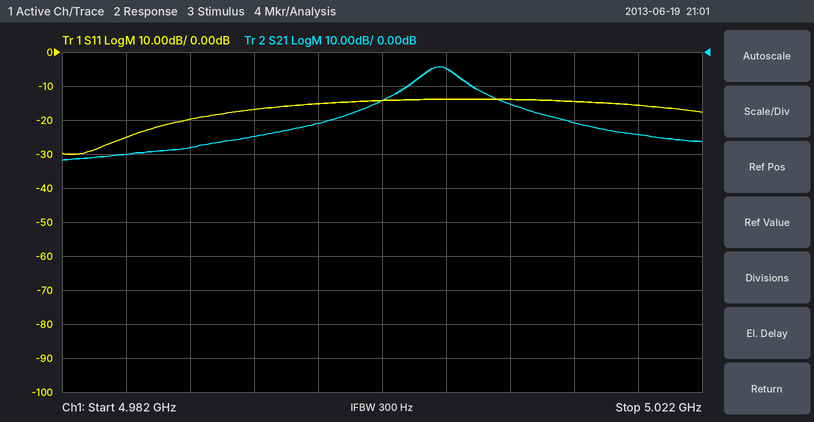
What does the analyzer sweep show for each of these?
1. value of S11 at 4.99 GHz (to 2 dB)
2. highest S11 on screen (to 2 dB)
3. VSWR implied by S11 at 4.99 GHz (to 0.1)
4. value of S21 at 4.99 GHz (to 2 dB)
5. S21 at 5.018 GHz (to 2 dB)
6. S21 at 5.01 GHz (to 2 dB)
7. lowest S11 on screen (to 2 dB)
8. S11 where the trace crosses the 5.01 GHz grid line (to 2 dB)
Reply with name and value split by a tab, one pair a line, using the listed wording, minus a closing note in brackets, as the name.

value of S11 at 4.99 GHz	-20 dB
highest S11 on screen	-14 dB
VSWR implied by S11 at 4.99 GHz	1.2
value of S21 at 4.99 GHz	-28 dB
S21 at 5.018 GHz	-24 dB
S21 at 5.01 GHz	-16 dB
lowest S11 on screen	-30 dB
S11 where the trace crosses the 5.01 GHz grid line	-14 dB
